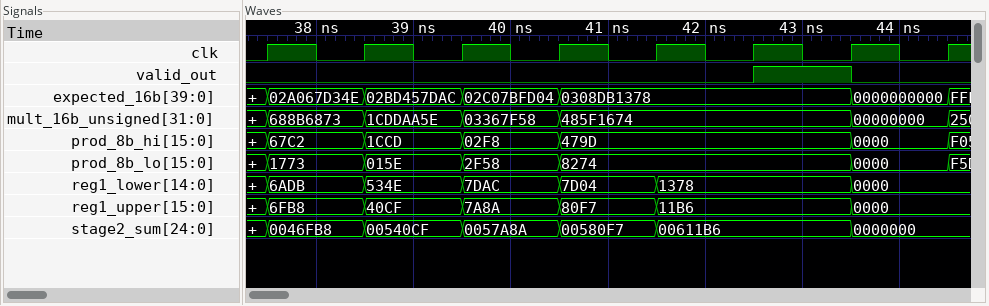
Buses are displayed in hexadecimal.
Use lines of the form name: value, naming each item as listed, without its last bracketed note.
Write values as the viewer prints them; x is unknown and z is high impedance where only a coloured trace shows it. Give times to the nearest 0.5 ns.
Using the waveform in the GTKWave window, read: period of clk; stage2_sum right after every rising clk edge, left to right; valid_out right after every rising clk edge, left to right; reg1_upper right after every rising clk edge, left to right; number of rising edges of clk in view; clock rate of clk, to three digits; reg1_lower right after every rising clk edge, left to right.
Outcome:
period of clk: 1 ns
stage2_sum right after every rising clk edge, left to right: 0046FB8, 00540CF, 0057A8A, 00580F7, 00611B6, 00611B6, 0000000, 0000000
valid_out right after every rising clk edge, left to right: 0 0 0 0 0 1 0 0
reg1_upper right after every rising clk edge, left to right: 6FB8, 40CF, 7A8A, 80F7, 11B6, 11B6, 0000, 0000
number of rising edges of clk in view: 8
clock rate of clk, to three digits: 1.00 GHz
reg1_lower right after every rising clk edge, left to right: 6ADB, 534E, 7DAC, 7D04, 1378, 1378, 0000, 0000
